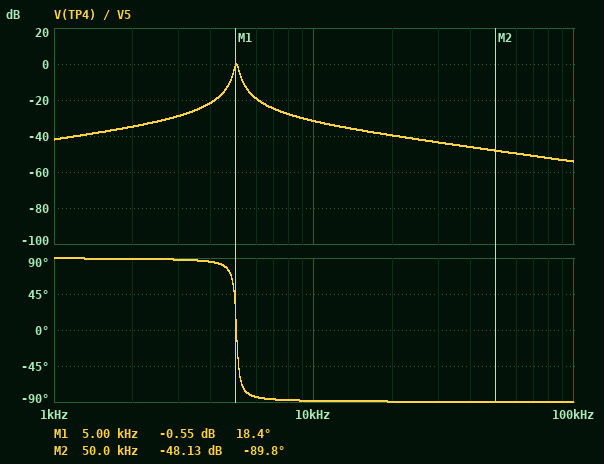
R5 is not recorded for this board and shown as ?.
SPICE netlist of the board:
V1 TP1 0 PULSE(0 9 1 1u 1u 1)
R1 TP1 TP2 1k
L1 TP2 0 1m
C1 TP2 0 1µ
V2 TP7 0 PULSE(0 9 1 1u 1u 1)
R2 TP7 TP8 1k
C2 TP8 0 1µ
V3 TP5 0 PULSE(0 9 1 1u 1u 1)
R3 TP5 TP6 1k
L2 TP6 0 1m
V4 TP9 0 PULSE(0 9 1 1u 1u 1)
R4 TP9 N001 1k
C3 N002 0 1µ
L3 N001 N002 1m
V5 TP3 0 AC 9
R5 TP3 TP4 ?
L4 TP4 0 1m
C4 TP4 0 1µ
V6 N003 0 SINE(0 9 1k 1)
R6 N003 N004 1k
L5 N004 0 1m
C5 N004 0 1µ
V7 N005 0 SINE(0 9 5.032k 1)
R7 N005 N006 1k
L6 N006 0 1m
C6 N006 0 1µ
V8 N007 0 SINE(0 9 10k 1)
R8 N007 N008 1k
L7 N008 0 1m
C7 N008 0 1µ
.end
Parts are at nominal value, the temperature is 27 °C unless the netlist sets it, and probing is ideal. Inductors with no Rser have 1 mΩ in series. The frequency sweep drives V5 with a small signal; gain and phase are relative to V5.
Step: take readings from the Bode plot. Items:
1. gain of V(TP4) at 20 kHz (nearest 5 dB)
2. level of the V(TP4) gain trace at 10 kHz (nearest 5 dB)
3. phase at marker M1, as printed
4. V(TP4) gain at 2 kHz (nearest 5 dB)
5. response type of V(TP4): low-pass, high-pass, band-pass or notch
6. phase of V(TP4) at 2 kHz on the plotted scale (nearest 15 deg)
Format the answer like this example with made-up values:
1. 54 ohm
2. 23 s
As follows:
1. -40 dB
2. -30 dB
3. 18.4 deg
4. -35 dB
5. band-pass
6. 90 deg
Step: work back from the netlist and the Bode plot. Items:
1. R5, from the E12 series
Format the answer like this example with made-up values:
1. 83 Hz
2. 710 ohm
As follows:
1. 820 Ω
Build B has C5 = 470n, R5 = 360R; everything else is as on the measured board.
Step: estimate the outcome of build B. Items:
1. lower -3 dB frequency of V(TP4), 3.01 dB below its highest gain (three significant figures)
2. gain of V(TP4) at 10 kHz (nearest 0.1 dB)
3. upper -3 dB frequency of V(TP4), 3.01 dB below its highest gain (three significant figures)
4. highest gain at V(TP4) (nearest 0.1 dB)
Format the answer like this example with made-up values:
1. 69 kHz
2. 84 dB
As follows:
1. 4.82 kHz
2. -24.6 dB
3. 5.26 kHz
4. 0 dB
